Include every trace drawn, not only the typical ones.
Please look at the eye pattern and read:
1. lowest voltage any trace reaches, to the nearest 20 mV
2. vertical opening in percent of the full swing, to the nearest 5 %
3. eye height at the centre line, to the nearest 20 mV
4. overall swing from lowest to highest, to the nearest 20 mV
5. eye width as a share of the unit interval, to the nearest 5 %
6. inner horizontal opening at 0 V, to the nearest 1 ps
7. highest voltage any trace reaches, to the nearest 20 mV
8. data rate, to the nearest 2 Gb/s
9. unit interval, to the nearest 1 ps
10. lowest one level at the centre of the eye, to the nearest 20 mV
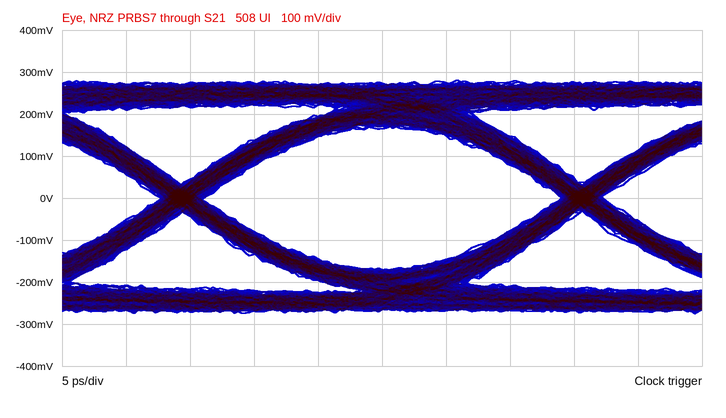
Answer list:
-280 mV
60 %
340 mV
560 mV
90 %
28 ps
280 mV
32 Gb/s
31 ps
160 mV
